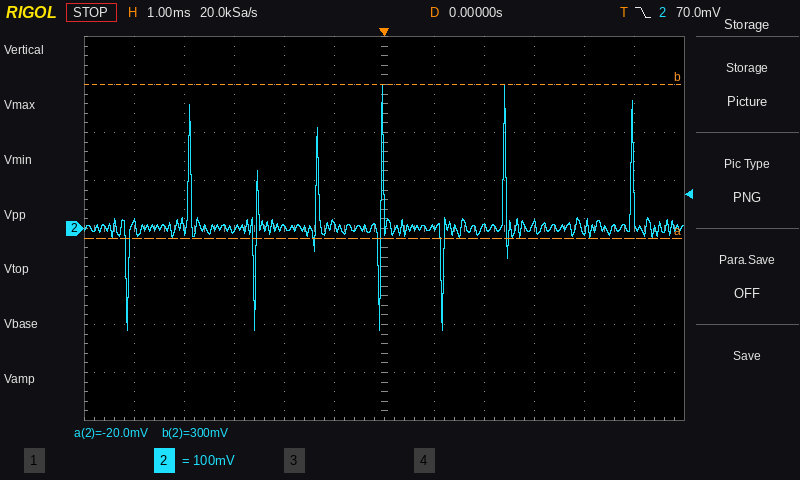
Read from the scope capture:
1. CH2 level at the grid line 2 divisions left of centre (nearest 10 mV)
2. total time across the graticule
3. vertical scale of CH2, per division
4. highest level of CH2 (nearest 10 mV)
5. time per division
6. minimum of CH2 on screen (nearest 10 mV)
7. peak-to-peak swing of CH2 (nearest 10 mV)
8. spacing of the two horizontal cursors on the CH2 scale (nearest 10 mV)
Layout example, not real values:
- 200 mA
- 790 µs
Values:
- 0 mV
- 12 ms
- 100 mV
- 300 mV
- 1 ms
- -210 mV
- 510 mV
- 320 mV
